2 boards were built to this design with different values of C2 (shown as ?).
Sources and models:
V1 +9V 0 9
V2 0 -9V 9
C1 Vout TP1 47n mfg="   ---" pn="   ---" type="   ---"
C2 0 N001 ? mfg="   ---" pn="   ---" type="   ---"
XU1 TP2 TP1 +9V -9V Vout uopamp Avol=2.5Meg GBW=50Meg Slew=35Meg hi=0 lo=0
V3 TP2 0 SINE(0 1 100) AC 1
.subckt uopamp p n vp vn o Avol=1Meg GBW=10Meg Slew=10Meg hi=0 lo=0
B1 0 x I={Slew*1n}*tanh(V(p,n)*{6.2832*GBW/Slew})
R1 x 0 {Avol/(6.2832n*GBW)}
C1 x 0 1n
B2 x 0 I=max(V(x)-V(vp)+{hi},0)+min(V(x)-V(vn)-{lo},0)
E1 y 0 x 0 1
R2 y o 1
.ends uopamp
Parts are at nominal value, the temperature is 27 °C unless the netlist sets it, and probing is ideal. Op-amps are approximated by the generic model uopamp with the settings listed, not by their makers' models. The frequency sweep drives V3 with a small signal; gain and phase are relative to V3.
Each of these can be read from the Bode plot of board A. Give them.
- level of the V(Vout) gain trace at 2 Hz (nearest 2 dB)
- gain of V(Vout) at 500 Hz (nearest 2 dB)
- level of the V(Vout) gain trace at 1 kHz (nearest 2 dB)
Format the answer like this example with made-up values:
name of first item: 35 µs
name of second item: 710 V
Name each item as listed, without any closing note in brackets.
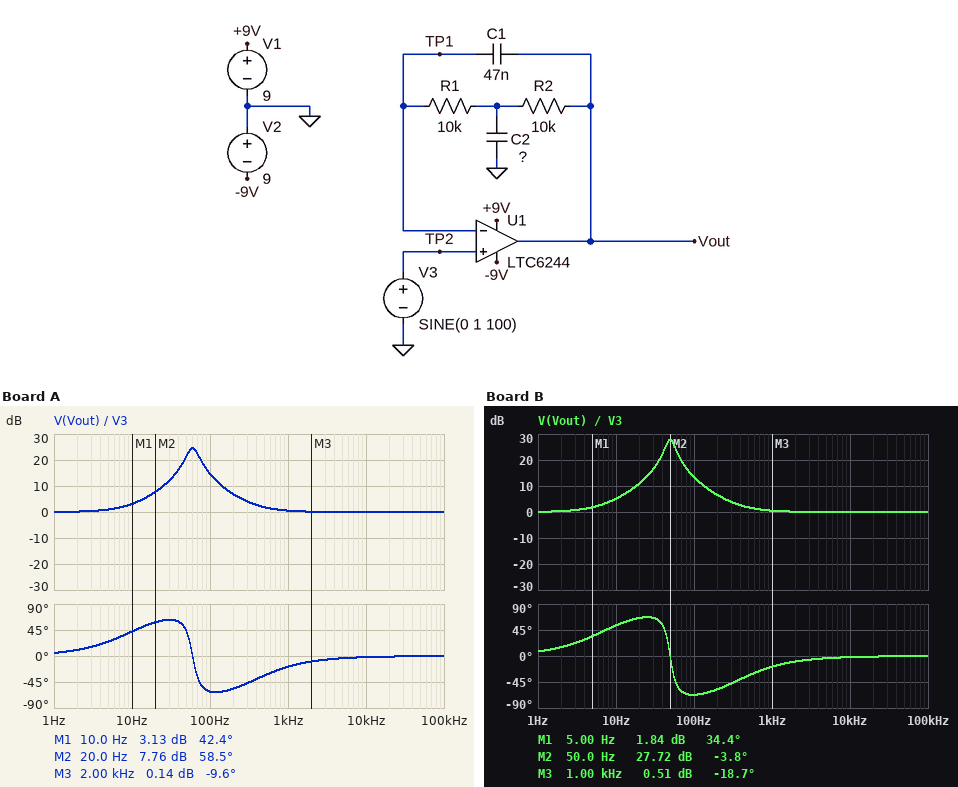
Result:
level of the V(Vout) gain trace at 2 Hz: 0 dB
gain of V(Vout) at 500 Hz: 2 dB
level of the V(Vout) gain trace at 1 kHz: 0 dB
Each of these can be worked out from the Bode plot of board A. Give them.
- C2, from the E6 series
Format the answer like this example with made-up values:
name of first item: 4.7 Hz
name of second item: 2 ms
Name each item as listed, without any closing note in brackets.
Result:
C2, from the E6 series: 1.5 µF
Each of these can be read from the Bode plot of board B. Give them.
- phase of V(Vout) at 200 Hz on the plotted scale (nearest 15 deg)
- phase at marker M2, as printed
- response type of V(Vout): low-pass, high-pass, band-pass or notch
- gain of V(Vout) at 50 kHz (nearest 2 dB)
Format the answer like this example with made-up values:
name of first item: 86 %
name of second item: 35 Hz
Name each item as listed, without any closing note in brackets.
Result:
phase of V(Vout) at 200 Hz on the plotted scale: -60 deg
phase at marker M2, as printed: -3.8 deg
response type of V(Vout): low-pass, high-pass, band-pass or notch: band-pass
gain of V(Vout) at 50 kHz: 0 dB
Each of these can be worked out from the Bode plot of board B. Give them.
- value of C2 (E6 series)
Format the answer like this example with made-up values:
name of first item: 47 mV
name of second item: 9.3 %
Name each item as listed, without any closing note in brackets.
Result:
value of C2: 2.2 µF
